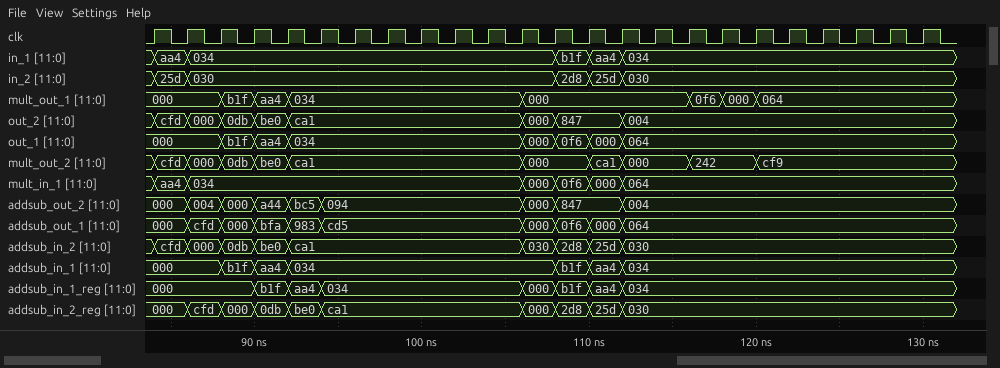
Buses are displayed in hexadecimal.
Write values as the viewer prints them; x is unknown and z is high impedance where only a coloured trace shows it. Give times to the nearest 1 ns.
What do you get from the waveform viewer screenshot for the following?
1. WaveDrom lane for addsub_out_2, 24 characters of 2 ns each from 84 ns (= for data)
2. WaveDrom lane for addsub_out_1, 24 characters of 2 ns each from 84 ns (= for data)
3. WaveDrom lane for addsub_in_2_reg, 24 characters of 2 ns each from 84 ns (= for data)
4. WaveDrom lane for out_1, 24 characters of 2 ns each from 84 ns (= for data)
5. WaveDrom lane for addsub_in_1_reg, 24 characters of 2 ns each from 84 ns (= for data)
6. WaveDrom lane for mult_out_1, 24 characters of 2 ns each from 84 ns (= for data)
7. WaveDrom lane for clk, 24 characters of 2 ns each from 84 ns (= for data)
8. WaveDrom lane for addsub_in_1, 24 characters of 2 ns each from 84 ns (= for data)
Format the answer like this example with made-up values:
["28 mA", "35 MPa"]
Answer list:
["{name: 'addsub_out_2', wave: '======.....==.=.........', data: '000 004 000 a44 bc5 094 000 847 004'}", "{name: 'addsub_out_1', wave: '======.....====.........', data: '000 cfd 000 bfa 983 cd5 000 0f6 000 064'}", "{name: 'addsub_in_2_reg', wave: '======.....====.........', data: '000 cfd 000 0db be0 ca1 000 2d8 25d 030'}", "{name: 'out_1', wave: '=.===......====.........', data: '000 b1f aa4 034 000 0f6 000 064'}", "{name: 'addsub_in_1_reg', wave: '=..===.....====.........', data: '000 b1f aa4 034 000 b1f aa4 034'}", "{name: 'mult_out_1', wave: '=.===......=....===.....', data: '000 b1f aa4 034 000 0f6 000 064'}", "{name: 'clk', wave: 'p.......................'}", "{name: 'addsub_in_1', wave: '=.===.......===.........', data: '000 b1f aa4 034 b1f aa4 034'}"]
